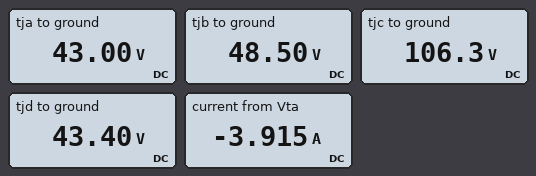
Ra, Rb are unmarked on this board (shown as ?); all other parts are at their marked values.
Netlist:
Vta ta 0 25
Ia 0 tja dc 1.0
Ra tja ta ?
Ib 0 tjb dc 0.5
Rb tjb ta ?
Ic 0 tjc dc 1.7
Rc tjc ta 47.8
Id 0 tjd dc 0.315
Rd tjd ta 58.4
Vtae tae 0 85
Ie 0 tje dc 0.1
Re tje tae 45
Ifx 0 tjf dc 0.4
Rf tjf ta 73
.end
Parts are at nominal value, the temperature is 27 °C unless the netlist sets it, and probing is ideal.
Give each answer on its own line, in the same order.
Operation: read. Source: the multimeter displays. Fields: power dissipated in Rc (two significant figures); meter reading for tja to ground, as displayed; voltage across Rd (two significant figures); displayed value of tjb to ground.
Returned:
140 W
43.00 V
18 V
48.50 V
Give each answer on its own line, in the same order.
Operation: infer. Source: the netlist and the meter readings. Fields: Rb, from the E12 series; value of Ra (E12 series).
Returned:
47 Ω
18 Ω
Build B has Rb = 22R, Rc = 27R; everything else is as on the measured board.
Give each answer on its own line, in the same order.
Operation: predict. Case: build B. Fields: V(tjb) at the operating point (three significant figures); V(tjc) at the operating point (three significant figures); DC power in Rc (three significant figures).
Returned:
36.0 V
70.9 V
78.0 W
